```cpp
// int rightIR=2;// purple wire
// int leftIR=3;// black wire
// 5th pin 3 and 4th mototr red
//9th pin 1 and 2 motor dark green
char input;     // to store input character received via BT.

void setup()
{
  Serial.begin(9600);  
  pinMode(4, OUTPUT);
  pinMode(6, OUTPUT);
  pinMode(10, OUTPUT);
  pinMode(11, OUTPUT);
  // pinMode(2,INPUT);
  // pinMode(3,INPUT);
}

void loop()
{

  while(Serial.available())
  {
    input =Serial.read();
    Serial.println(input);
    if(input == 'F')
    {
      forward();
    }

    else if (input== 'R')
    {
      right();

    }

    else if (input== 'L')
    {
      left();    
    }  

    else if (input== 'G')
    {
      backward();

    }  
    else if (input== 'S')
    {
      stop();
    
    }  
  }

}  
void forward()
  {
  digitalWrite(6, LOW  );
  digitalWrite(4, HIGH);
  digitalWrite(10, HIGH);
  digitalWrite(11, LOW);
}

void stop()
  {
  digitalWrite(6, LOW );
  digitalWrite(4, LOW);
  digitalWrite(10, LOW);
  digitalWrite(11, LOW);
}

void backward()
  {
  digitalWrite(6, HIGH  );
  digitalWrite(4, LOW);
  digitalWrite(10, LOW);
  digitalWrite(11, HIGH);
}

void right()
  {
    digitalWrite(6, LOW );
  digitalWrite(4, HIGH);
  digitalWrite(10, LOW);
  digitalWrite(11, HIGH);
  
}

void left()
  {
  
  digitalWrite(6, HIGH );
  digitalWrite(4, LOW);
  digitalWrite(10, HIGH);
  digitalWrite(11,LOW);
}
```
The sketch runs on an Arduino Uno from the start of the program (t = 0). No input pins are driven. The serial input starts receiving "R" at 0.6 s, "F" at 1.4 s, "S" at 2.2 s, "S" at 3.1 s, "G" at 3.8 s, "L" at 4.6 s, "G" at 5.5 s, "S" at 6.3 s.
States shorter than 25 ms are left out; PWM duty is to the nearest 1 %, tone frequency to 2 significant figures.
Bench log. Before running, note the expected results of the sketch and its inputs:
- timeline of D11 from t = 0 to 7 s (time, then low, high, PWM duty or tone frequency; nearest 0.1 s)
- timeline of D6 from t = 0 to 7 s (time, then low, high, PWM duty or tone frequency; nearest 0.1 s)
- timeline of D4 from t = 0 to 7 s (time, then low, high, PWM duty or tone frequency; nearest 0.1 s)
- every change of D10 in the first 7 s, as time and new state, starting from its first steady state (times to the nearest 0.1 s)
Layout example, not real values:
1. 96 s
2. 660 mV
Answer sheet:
1. 0 s low; 0.6 s high; 1.4 s low; 3.8 s high; 4.6 s low; 5.5 s high; 6.3 s low
2. 0 s low; 3.8 s high; 6.3 s low
3. 0 s low; 0.6 s high; 2.2 s low
4. 0 s low; 1.4 s high; 2.2 s low; 4.6 s high; 5.5 s low
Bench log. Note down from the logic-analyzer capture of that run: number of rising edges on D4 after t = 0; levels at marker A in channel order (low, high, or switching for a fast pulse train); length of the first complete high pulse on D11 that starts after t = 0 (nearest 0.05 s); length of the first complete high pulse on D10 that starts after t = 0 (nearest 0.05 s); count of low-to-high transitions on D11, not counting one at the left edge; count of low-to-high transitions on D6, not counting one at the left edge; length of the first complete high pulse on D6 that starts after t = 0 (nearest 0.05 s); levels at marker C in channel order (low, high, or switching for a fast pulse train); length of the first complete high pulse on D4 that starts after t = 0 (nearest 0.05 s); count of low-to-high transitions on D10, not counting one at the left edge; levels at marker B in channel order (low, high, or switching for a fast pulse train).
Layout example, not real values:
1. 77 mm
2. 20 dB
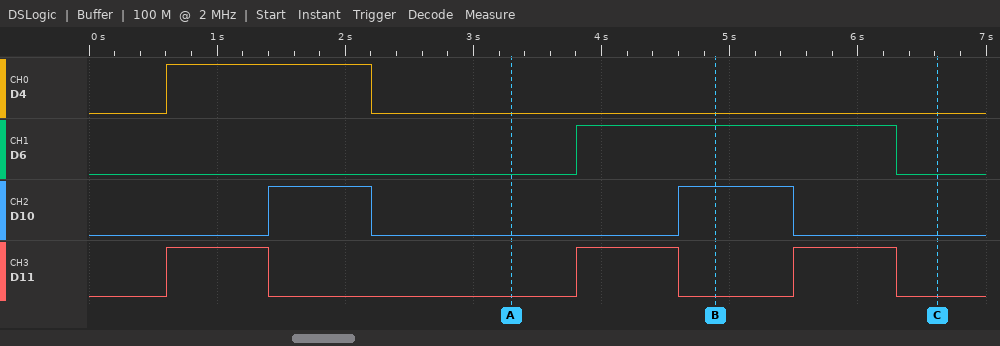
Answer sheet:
1. 1
2. D4 low, D6 low, D10 low, D11 low
3. 0.80 s
4. 0.80 s
5. 3
6. 1
7. 2.50 s
8. D4 low, D6 low, D10 low, D11 low
9. 1.60 s
10. 2
11. D4 low, D6 high, D10 high, D11 low
